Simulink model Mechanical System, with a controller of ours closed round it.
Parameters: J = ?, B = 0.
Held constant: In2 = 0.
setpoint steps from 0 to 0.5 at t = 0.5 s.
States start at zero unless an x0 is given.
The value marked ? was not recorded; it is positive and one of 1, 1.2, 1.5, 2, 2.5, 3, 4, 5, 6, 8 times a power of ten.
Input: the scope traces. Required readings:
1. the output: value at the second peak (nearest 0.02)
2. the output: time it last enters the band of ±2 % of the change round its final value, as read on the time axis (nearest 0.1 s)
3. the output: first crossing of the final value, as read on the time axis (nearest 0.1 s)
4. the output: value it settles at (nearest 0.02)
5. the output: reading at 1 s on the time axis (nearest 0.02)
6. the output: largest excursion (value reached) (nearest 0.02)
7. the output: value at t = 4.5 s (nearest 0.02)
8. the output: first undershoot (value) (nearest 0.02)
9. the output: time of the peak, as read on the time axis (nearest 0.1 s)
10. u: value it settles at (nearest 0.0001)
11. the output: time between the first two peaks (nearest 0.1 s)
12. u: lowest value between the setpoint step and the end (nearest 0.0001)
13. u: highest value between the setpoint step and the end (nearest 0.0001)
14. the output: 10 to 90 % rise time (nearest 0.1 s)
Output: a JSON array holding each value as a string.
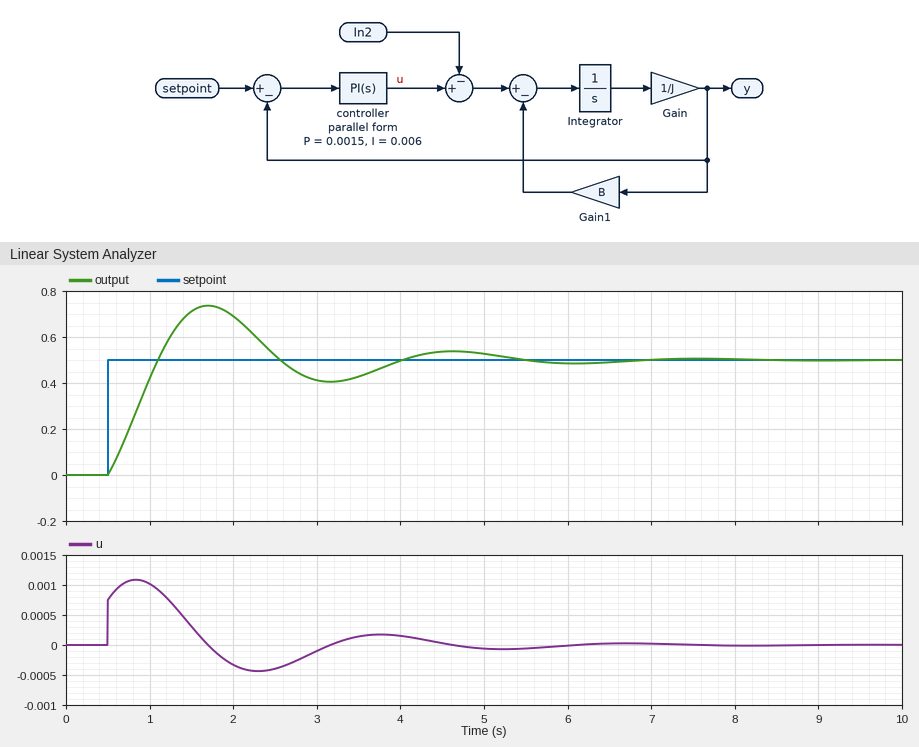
["0.54", "6.5 s", "1.1 s", "0.50", "0.42", "0.74", "0.54", "0.40", "1.7 s", "0.0000", "2.9 s", "-0.0004", "0.0011", "0.5 s"]
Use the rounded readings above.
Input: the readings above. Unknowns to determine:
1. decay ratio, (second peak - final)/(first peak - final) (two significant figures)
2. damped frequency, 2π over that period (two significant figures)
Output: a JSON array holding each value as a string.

["0.17", "2.2 rad/s"]
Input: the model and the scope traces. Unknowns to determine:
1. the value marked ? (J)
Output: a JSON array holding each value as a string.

["0.0012"]
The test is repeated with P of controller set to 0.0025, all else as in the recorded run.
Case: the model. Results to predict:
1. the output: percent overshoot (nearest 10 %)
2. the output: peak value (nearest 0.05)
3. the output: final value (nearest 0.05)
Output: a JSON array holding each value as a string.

["30 %", "0.65", "0.50"]
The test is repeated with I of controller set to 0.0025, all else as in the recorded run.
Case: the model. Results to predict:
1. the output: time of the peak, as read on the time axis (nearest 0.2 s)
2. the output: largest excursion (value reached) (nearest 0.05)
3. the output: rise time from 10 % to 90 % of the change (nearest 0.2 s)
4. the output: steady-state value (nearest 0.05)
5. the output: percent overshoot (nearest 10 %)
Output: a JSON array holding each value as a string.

["2.2 s", "0.65", "0.6 s", "0.50", "30 %"]
